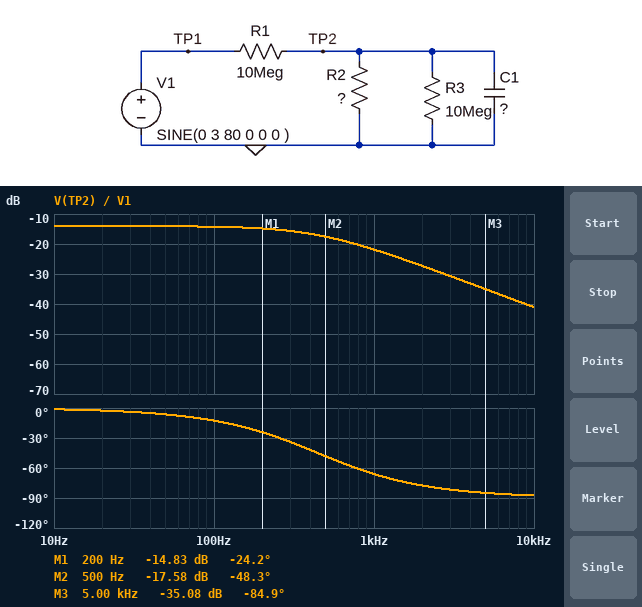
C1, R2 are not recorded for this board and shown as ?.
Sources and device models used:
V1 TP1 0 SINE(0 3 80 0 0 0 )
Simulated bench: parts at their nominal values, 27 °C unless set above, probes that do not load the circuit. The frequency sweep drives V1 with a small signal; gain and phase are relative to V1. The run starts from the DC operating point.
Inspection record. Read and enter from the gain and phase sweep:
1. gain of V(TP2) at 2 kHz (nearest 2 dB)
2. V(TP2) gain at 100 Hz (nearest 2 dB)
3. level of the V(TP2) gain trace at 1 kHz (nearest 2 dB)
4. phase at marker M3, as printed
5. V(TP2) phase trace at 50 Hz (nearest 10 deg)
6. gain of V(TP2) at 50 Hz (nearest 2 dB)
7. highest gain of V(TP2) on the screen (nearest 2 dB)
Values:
-28 dB
-14 dB
-22 dB
-84.9 deg
-10 deg
-14 dB
-14 dB
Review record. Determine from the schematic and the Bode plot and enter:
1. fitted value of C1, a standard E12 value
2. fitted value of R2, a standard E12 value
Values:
180 pF
3.3 MΩ
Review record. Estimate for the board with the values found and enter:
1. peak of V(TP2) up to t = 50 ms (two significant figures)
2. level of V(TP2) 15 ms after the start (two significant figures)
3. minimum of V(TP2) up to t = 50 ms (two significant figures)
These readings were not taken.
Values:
590 mV
520 mV
-590 mV
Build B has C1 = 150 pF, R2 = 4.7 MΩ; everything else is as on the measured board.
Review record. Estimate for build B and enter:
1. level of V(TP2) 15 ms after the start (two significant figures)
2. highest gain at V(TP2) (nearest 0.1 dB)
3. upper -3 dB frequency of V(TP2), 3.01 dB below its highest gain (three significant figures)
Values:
630 mV
-12.3 dB
438 Hz
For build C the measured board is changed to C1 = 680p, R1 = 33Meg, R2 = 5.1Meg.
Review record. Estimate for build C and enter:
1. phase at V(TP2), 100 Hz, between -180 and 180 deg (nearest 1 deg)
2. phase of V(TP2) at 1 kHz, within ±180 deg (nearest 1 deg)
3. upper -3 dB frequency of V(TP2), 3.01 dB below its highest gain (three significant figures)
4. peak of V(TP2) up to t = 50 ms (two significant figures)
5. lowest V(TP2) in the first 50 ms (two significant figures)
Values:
-53 deg
-86 deg
76.4 Hz
210 mV
-190 mV
